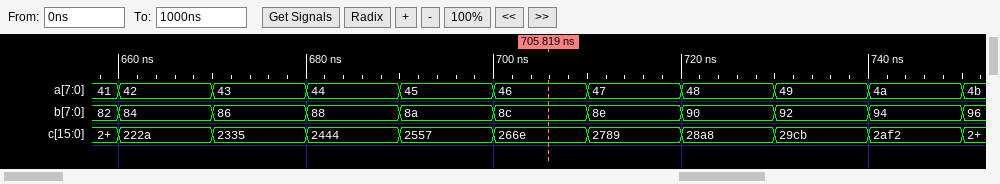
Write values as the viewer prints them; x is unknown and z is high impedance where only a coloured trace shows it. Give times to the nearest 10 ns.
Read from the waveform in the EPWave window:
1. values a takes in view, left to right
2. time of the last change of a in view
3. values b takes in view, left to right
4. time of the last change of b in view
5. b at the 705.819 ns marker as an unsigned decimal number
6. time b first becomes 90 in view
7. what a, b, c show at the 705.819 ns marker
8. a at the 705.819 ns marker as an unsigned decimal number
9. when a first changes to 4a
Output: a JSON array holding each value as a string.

["41, 42, 43, 44, 45, 46, 47, 48, 49, 4a, 4b", "750 ns", "82, 84, 86, 88, 8a, 8c, 8e, 90, 92, 94, 96", "750 ns", "140", "720 ns", "a=46, b=8c, c=266e", "70", "740 ns"]
